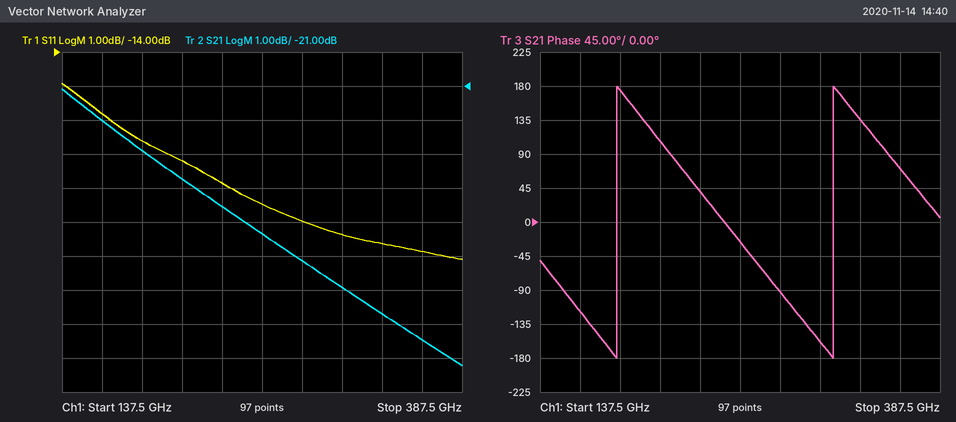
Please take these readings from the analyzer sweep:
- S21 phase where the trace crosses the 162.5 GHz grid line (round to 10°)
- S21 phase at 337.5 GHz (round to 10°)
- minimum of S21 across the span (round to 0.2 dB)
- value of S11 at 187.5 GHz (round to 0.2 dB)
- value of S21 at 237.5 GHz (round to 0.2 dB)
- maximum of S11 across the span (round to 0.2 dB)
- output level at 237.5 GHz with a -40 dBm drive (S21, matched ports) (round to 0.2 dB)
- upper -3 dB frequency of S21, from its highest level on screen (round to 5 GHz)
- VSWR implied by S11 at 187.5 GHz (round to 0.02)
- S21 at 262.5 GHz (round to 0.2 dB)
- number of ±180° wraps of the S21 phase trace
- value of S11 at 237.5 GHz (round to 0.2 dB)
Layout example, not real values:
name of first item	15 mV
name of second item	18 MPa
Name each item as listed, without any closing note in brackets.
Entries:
S21 phase where the trace crosses the 162.5 GHz grid line	-120°
S21 phase at 337.5 GHz	140°
minimum of S21 across the span	-29.2 dB
value of S11 at 187.5 GHz	-16.6 dB
value of S21 at 237.5 GHz	-24.6 dB
maximum of S11 across the span	-15.0 dB
output level at 237.5 GHz with a -40 dBm drive (S21, matched ports)	-64.6 dBm
upper -3 dB frequency of S21, from its highest level on screen	225 GHz
VSWR implied by S11 at 187.5 GHz	1.34
S21 at 262.5 GHz	-25.4 dB
number of ±180° wraps of the S21 phase trace	2
value of S11 at 237.5 GHz	-17.8 dB
